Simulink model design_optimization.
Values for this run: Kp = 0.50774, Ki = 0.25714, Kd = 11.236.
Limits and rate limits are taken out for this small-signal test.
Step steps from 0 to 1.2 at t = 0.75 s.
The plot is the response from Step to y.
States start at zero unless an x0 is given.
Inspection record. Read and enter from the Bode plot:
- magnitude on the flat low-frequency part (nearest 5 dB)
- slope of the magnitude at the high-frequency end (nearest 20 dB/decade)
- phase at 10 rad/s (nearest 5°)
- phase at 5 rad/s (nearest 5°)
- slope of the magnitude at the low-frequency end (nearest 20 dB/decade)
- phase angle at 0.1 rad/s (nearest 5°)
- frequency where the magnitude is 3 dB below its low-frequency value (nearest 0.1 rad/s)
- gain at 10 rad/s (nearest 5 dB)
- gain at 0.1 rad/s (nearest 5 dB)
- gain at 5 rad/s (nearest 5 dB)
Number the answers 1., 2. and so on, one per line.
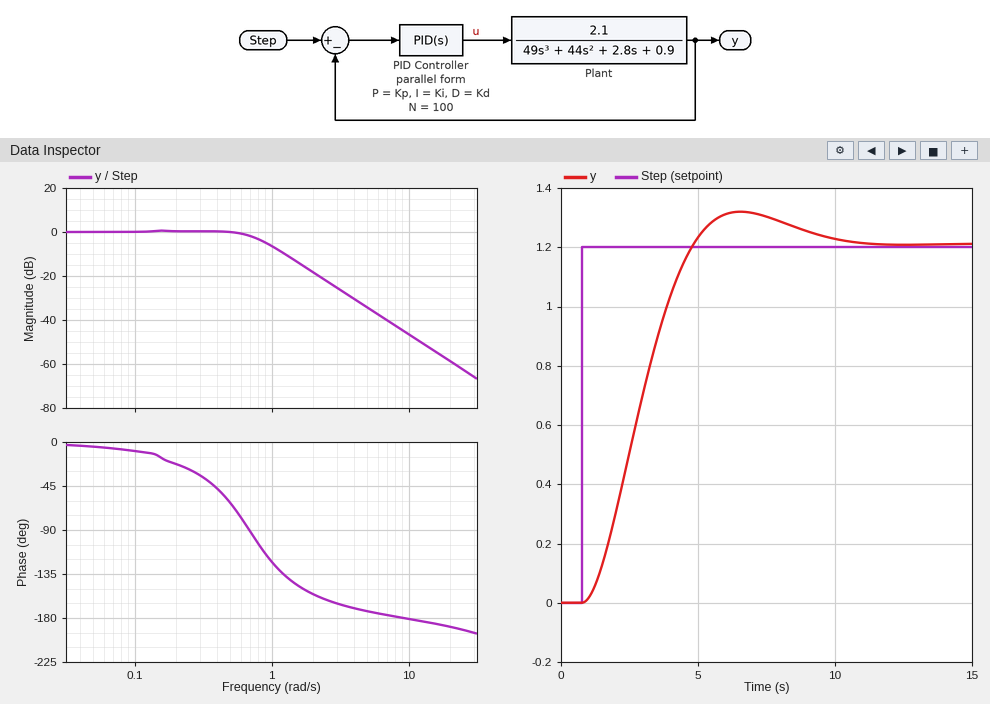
1. 0 dB
2. -40 dB/decade
3. -180°
4. -175°
5. 0 dB/decade
6. -10°
7. 0.8 rad/s
8. -45 dB
9. 0 dB
10. -35 dB
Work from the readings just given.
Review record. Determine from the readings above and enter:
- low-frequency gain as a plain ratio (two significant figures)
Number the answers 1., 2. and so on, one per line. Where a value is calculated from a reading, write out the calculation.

1. 10^(0 / 20) = 1.0
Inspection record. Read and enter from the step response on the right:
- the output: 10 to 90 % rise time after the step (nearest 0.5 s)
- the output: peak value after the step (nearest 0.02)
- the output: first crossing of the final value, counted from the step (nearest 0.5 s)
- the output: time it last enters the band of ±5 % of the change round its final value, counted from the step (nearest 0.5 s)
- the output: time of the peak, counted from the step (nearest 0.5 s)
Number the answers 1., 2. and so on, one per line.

1. 2.5 s
2. 1.32
3. 4.0 s
4. 8.0 s
5. 6.0 s
